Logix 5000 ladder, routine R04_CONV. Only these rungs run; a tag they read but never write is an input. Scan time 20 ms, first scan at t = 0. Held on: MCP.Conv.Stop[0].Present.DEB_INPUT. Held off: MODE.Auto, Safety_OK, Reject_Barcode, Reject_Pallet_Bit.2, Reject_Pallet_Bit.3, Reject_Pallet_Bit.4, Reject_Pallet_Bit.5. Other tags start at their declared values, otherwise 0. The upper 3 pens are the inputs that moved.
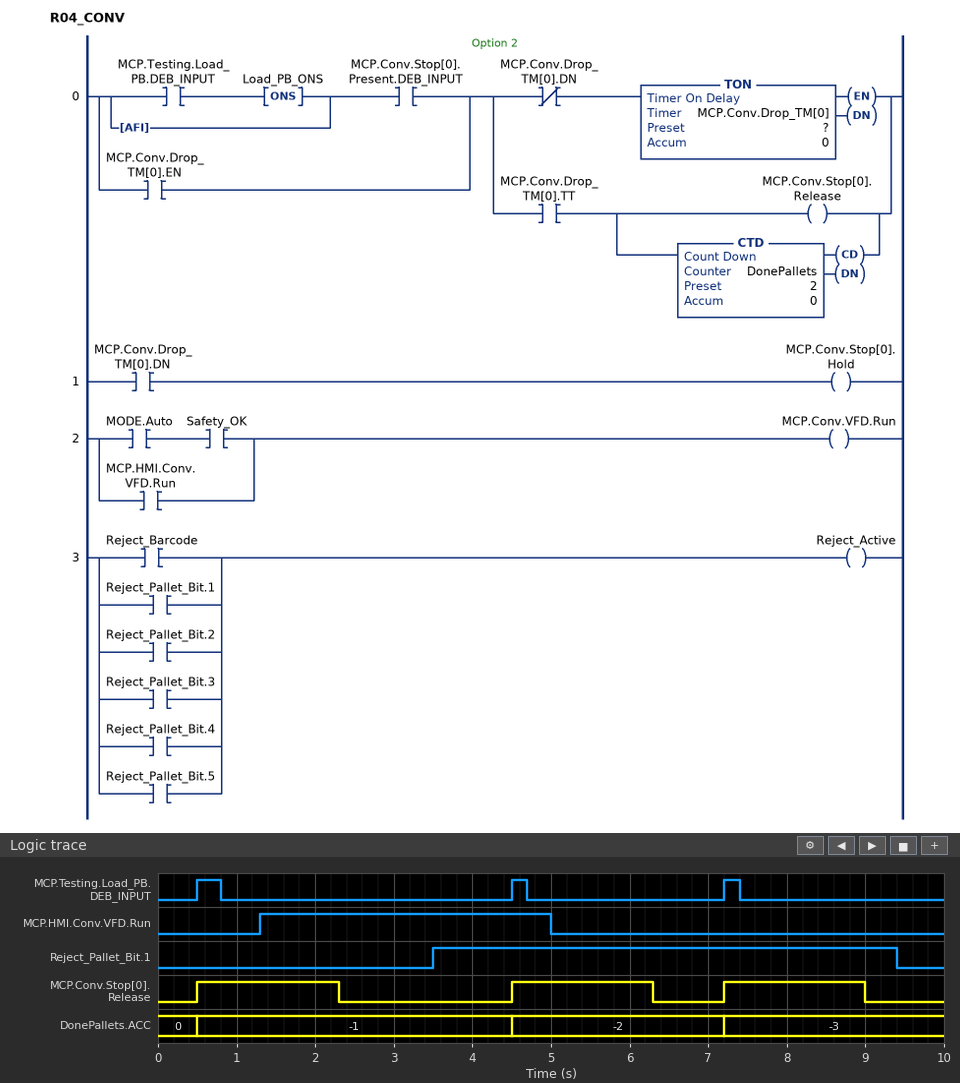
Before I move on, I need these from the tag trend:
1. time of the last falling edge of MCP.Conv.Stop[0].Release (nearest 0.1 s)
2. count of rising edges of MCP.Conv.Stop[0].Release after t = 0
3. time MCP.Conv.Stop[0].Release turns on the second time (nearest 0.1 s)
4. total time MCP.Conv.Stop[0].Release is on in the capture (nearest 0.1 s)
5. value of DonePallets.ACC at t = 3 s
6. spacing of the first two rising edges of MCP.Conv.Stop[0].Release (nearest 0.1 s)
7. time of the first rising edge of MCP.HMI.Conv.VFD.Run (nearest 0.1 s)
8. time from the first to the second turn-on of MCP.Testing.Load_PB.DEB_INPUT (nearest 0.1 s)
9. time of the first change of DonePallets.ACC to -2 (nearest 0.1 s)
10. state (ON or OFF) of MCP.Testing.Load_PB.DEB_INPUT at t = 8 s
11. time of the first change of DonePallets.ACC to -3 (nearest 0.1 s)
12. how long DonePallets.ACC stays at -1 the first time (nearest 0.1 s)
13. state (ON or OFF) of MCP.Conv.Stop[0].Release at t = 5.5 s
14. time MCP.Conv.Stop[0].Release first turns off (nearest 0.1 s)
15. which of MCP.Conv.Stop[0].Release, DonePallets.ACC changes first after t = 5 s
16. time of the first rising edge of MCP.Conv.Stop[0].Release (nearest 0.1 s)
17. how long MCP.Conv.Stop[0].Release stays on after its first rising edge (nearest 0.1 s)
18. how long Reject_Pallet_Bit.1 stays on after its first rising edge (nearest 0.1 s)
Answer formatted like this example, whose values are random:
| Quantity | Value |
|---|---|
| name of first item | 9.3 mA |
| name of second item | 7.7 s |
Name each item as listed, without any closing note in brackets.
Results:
| Quantity | Value |
|---|---|
| time of the last falling edge of MCP.Conv.Stop[0].Release | 9.0 s |
| count of rising edges of MCP.Conv.Stop[0].Release after t = 0 | 3 |
| time MCP.Conv.Stop[0].Release turns on the second time | 4.5 s |
| total time MCP.Conv.Stop[0].Release is on in the capture | 5.4 s |
| value of DonePallets.ACC at t = 3 s | -1 |
| spacing of the first two rising edges of MCP.Conv.Stop[0].Release | 4.0 s |
| time of the first rising edge of MCP.HMI.Conv.VFD.Run | 1.3 s |
| time from the first to the second turn-on of MCP.Testing.Load_PB.DEB_INPUT | 4.0 s |
| time of the first change of DonePallets.ACC to -2 | 4.5 s |
| state (ON or OFF) of MCP.Testing.Load_PB.DEB_INPUT at t = 8 s | OFF |
| time of the first change of DonePallets.ACC to -3 | 7.2 s |
| how long DonePallets.ACC stays at -1 the first time | 4.0 s |
| state (ON or OFF) of MCP.Conv.Stop[0].Release at t = 5.5 s | ON |
| time MCP.Conv.Stop[0].Release first turns off | 2.3 s |
| which of MCP.Conv.Stop[0].Release, DonePallets.ACC changes first after t = 5 s | MCP.Conv.Stop[0].Release |
| time of the first rising edge of MCP.Conv.Stop[0].Release | 0.5 s |
| how long MCP.Conv.Stop[0].Release stays on after its first rising edge | 1.8 s |
| how long Reject_Pallet_Bit.1 stays on after its first rising edge | 5.9 s |
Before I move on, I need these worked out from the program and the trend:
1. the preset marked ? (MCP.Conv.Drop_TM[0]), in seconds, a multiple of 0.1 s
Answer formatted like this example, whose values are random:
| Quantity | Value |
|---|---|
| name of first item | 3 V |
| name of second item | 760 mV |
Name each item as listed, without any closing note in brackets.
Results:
| Quantity | Value |
|---|---|
| the preset marked ? (MCP.Conv.Drop_TM[0]), in seconds, a multiple of 0.1 s | 1.8 s |
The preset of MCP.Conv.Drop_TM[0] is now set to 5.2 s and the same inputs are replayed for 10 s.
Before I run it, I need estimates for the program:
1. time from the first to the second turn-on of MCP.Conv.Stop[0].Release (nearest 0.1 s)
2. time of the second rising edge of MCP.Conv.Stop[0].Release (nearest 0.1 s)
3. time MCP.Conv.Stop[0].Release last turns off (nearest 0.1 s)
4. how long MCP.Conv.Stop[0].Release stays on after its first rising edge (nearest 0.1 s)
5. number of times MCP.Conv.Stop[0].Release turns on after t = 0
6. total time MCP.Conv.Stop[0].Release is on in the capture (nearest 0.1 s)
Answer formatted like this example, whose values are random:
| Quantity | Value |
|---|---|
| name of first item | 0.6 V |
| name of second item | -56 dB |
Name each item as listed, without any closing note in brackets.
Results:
| Quantity | Value |
|---|---|
| time from the first to the second turn-on of MCP.Conv.Stop[0].Release | 6.7 s |
| time of the second rising edge of MCP.Conv.Stop[0].Release | 7.2 s |
| time MCP.Conv.Stop[0].Release last turns off | 5.7 s |
| how long MCP.Conv.Stop[0].Release stays on after its first rising edge | 5.2 s |
| number of times MCP.Conv.Stop[0].Release turns on after t = 0 | 2 |
| total time MCP.Conv.Stop[0].Release is on in the capture | 8.0 s |
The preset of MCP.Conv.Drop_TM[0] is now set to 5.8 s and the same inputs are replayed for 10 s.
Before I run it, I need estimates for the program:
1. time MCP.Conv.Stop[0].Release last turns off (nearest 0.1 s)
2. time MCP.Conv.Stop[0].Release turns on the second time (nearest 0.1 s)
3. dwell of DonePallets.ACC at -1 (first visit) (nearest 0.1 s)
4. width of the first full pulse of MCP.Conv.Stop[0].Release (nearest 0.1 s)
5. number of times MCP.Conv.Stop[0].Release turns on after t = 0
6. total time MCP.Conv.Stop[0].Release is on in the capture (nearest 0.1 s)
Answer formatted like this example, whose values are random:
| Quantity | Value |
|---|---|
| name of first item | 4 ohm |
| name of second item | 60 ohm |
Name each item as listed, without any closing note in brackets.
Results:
| Quantity | Value |
|---|---|
| time MCP.Conv.Stop[0].Release last turns off | 6.3 s |
| time MCP.Conv.Stop[0].Release turns on the second time | 7.2 s |
| dwell of DonePallets.ACC at -1 (first visit) | 6.7 s |
| width of the first full pulse of MCP.Conv.Stop[0].Release | 5.8 s |
| number of times MCP.Conv.Stop[0].Release turns on after t = 0 | 2 |
| total time MCP.Conv.Stop[0].Release is on in the capture | 8.6 s |
